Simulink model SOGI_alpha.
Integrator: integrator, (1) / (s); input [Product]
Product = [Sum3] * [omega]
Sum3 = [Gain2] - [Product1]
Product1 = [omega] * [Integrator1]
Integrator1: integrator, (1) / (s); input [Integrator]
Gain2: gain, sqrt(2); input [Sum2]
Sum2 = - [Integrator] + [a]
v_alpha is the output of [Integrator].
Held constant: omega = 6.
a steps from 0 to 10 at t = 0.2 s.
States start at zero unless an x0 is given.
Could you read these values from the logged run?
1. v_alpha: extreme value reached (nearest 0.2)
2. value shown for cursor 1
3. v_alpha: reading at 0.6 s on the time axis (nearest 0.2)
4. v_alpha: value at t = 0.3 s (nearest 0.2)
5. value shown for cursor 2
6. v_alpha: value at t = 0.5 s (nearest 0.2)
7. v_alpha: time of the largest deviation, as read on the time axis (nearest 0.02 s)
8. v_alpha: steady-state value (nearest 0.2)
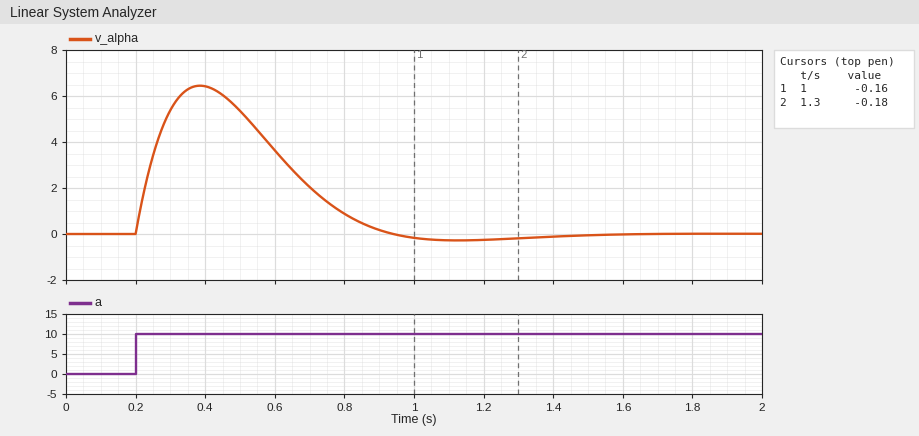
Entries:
6.4
-0.16
3.6
5.4
-0.18
5.4
0.38 s
0.0
